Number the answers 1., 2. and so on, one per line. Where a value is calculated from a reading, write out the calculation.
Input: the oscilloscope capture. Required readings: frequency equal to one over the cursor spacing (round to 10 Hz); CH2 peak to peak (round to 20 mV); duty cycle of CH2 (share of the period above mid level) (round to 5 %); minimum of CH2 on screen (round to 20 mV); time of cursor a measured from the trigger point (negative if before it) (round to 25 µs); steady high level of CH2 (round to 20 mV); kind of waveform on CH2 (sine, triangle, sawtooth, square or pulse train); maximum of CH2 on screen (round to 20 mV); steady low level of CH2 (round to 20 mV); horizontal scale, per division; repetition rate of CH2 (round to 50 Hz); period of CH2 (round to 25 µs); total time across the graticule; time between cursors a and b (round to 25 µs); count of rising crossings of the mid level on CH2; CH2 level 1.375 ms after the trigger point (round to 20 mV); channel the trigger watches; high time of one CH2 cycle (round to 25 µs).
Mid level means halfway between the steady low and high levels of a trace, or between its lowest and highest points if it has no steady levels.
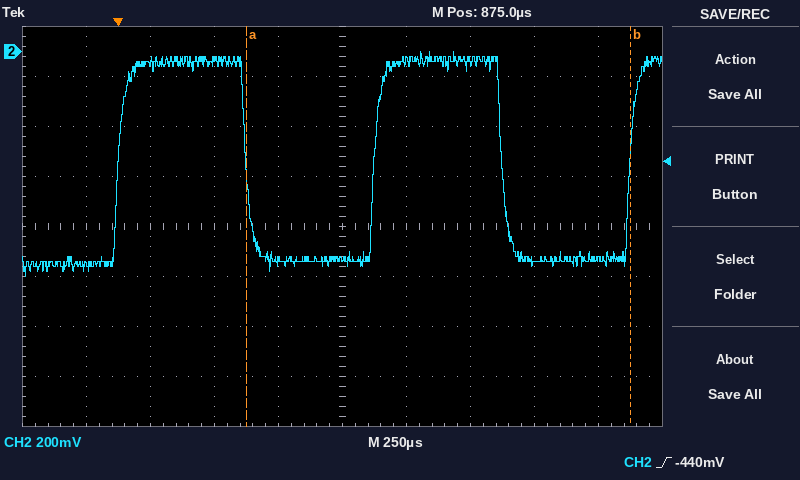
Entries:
1. 1 / 1.500 ms ≈ 670 Hz
2. 0 mV − (-900 mV) = 900 mV
3. 500 µs / 1.000 ms ≈ 50 %
4. -900 mV
5. +500 µs
6. -40 mV
7. square
8. 0 mV
9. -840 mV
10. 250 µs
11. 1 / 1.000 ms ≈ 1.00 kHz
12. 1.000 ms
13. 2.5 ms
14. 1.500 ms
15. 3
16. -40 mV
17. CH2
18. 500 µs
